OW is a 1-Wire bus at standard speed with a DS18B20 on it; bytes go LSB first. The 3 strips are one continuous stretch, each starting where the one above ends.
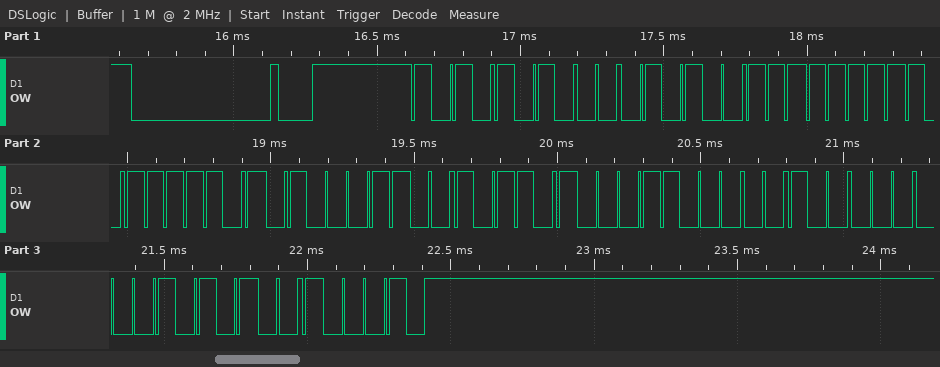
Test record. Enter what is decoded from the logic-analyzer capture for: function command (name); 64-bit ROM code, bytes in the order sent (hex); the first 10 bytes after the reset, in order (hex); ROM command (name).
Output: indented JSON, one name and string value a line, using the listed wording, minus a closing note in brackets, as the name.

{
  "function command": "Convert T",
  "64-bit ROM code, bytes in the order sent": "28 FF 7D C5 B4 18 04 A8",
  "the first 10 bytes after the reset, in order": "55 28 FF 7D C5 B4 18 04 A8 44",
  "ROM command": "Match ROM"
}
